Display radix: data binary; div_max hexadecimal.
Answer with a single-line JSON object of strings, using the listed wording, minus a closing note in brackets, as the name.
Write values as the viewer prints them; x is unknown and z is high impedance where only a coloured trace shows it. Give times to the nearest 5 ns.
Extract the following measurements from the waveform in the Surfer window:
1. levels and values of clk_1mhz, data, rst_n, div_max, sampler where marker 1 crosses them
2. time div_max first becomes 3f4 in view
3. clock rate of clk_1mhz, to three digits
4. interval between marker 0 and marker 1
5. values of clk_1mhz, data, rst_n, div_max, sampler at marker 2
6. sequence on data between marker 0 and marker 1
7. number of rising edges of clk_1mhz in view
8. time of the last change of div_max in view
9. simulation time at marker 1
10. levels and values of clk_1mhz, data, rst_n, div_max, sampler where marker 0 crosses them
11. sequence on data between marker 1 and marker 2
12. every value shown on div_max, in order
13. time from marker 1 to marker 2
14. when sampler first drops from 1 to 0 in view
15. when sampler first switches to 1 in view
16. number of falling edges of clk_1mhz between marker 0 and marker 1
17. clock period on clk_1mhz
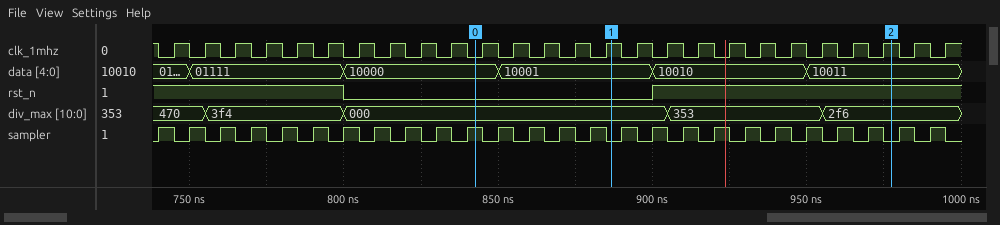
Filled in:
{"levels and values of clk_1mhz, data, rst_n, div_max, sampler where marker 1 crosses them": "clk_1mhz=1, data=10001, rst_n=0, div_max=000, sampler=0", "time div_max first becomes 3f4 in view": "755 ns", "clock rate of clk_1mhz, to three digits": "100 MHz", "interval between marker 0 and marker 1": "45 ns", "values of clk_1mhz, data, rst_n, div_max, sampler at marker 2": "clk_1mhz=1, data=10011, rst_n=1, div_max=2f6, sampler=0", "sequence on data between marker 0 and marker 1": "10000, 10001", "number of rising edges of clk_1mhz in view": "26", "time of the last change of div_max in view": "955 ns", "simulation time at marker 1": "885 ns", "levels and values of clk_1mhz, data, rst_n, div_max, sampler where marker 0 crosses them": "clk_1mhz=0, data=10000, rst_n=0, div_max=000, sampler=1", "sequence on data between marker 1 and marker 2": "10001, 10010, 10011", "every value shown on div_max, in order": "470, 3f4, 000, 353, 2f6", "time from marker 1 to marker 2": "90 ns", "when sampler first drops from 1 to 0 in view": "745 ns", "when sampler first switches to 1 in view": "740 ns", "number of falling edges of clk_1mhz between marker 0 and marker 1": "4", "clock period on clk_1mhz": "10 ns"}
